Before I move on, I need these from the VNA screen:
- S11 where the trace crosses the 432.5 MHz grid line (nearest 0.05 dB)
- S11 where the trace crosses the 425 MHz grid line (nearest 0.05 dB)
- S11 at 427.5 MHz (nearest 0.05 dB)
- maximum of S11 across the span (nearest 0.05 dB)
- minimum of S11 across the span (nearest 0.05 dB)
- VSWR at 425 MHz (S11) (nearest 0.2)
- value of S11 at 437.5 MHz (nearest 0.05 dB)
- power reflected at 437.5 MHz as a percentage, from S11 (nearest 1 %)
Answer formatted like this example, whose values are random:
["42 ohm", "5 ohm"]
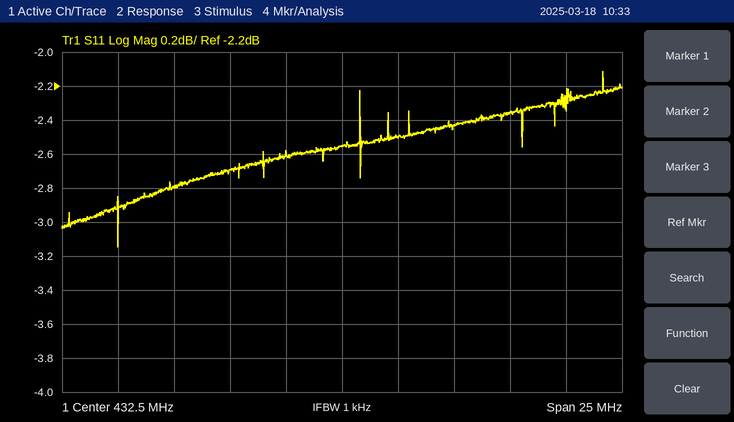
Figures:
["-2.55 dB", "-2.80 dB", "-2.70 dB", "-2.10 dB", "-3.15 dB", "6.2", "-2.45 dB", "57 %"]
